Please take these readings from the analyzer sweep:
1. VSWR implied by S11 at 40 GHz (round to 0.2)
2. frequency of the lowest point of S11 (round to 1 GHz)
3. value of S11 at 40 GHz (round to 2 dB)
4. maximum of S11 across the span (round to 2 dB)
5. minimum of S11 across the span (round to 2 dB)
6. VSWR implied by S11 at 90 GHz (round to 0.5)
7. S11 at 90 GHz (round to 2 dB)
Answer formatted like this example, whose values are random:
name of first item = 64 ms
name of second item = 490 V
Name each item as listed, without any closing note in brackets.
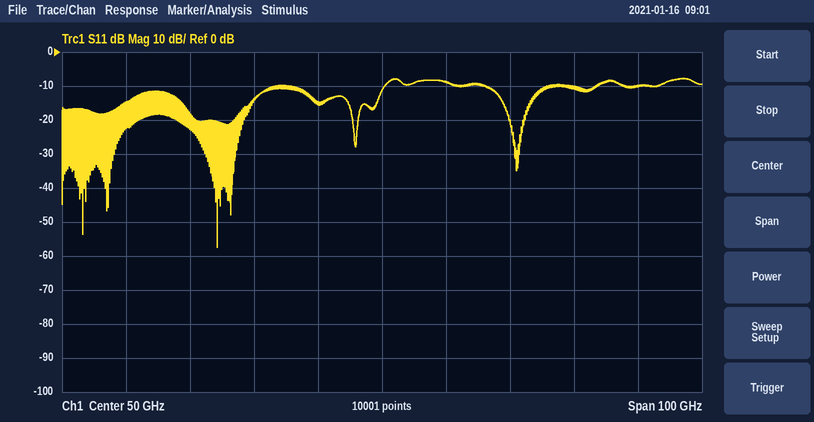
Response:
VSWR implied by S11 at 40 GHz = 1.4
frequency of the lowest point of S11 = 24 GHz
value of S11 at 40 GHz = -16 dB
maximum of S11 across the span = -8 dB
minimum of S11 across the span = -58 dB
VSWR implied by S11 at 90 GHz = 2.0
S11 at 90 GHz = -10 dB
